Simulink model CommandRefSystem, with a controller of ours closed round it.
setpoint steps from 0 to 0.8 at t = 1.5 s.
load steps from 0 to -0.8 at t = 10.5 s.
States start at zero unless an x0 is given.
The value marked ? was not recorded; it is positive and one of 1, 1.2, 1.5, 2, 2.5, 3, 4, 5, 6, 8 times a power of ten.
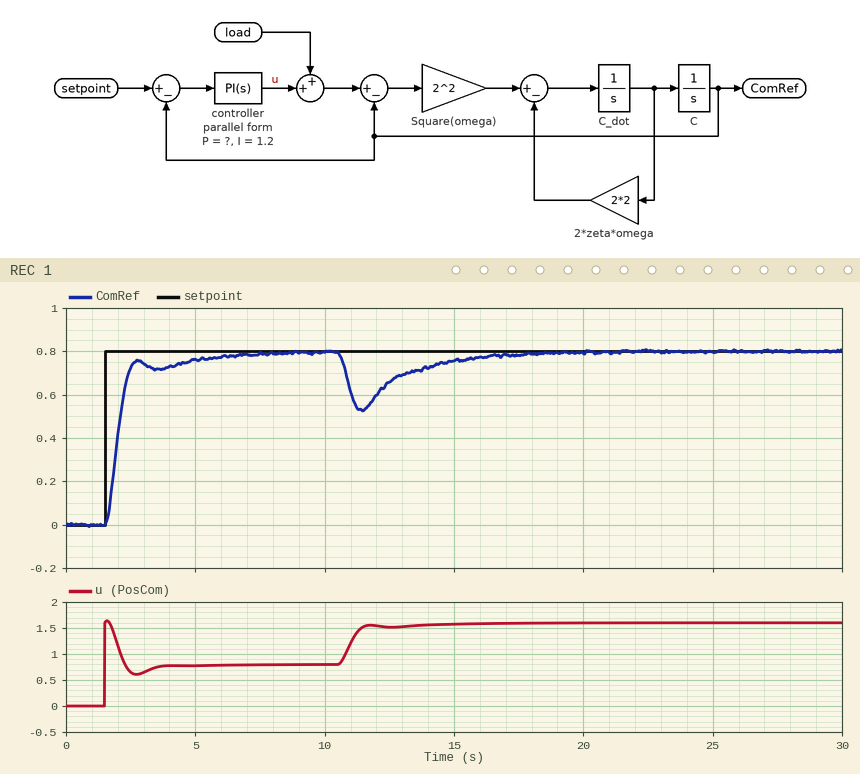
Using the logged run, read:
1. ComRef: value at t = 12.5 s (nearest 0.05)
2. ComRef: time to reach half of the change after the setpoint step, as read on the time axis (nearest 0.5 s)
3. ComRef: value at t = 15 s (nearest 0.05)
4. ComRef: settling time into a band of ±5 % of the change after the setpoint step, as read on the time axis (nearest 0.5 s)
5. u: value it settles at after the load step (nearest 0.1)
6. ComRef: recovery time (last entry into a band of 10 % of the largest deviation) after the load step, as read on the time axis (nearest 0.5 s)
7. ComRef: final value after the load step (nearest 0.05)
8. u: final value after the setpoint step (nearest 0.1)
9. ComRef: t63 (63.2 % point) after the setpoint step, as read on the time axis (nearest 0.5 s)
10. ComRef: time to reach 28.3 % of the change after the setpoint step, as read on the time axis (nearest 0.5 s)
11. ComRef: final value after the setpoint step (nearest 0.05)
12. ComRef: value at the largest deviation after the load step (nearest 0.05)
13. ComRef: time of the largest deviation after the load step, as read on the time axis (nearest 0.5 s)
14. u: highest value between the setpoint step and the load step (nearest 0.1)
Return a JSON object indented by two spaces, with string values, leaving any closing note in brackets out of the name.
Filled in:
{
  "ComRef: value at t = 12.5 s": "0.65",
  "ComRef: time to reach half of the change after the setpoint step, as read on the time axis": "2.0 s",
  "ComRef: value at t = 15 s": "0.75",
  "ComRef: settling time into a band of ±5 % of the change after the setpoint step, as read on the time axis": "5.0 s",
  "u: value it settles at after the load step": "1.6",
  "ComRef: recovery time (last entry into a band of 10 % of the largest deviation) after the load step, as read on the time axis": "16.0 s",
  "ComRef: final value after the load step": "0.80",
  "u: final value after the setpoint step": "0.8",
  "ComRef: t63 (63.2 % point) after the setpoint step, as read on the time axis": "2.0 s",
  "ComRef: time to reach 28.3 % of the change after the setpoint step, as read on the time axis": "2.0 s",
  "ComRef: final value after the setpoint step": "0.80",
  "ComRef: value at the largest deviation after the load step": "0.55",
  "ComRef: time of the largest deviation after the load step, as read on the time axis": "11.5 s",
  "u: highest value between the setpoint step and the load step": "1.6"
}
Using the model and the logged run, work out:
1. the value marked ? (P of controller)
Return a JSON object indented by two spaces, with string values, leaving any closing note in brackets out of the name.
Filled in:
{
  "the value marked ?": "2"
}
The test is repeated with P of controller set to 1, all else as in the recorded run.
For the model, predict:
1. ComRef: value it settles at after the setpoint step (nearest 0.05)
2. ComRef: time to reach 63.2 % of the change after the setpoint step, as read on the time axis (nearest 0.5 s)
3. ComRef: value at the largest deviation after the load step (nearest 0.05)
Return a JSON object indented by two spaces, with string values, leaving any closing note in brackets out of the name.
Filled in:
{
  "ComRef: value it settles at after the setpoint step": "0.80",
  "ComRef: time to reach 63.2 % of the change after the setpoint step, as read on the time axis": "2.5 s",
  "ComRef: value at the largest deviation after the load step": "0.45"
}
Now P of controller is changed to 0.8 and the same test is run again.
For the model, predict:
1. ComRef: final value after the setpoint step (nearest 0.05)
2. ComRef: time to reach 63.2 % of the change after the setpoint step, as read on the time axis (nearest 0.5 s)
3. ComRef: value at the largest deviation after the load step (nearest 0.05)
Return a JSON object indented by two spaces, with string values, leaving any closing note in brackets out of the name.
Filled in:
{
  "ComRef: final value after the setpoint step": "0.80",
  "ComRef: time to reach 63.2 % of the change after the setpoint step, as read on the time axis": "2.5 s",
  "ComRef: value at the largest deviation after the load step": "0.45"
}
